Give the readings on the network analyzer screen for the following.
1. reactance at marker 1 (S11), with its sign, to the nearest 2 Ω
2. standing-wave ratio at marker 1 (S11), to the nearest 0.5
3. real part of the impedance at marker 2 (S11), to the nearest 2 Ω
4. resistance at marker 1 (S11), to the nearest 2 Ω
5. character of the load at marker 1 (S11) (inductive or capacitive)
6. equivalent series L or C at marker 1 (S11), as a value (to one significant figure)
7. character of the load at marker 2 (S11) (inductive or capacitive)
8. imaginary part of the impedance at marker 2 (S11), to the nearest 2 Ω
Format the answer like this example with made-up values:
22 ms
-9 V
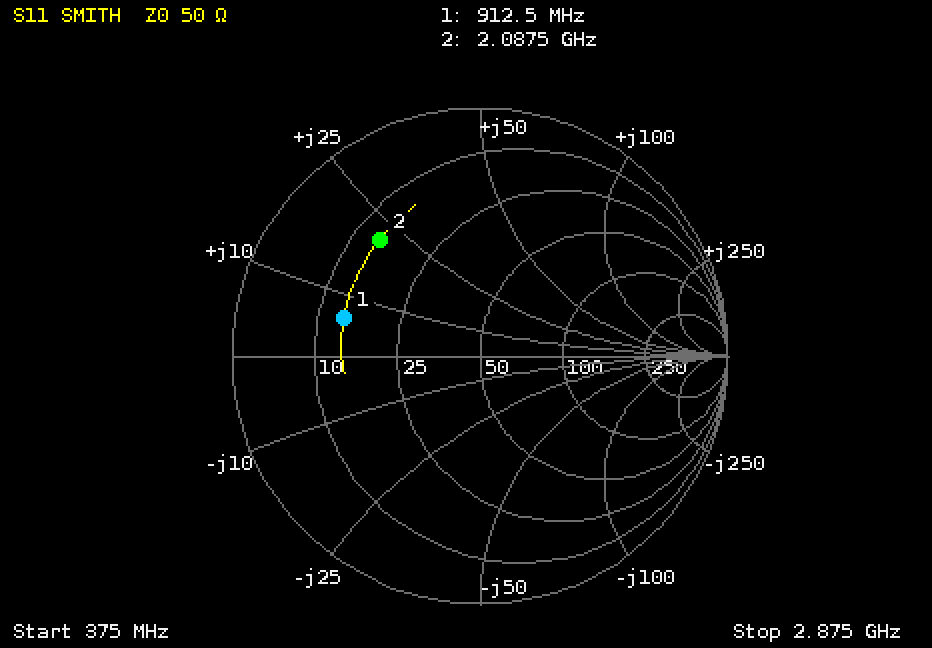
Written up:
+6 Ω
3.5
14 Ω
14 Ω
inductive
1 nH
inductive
+22 Ω
